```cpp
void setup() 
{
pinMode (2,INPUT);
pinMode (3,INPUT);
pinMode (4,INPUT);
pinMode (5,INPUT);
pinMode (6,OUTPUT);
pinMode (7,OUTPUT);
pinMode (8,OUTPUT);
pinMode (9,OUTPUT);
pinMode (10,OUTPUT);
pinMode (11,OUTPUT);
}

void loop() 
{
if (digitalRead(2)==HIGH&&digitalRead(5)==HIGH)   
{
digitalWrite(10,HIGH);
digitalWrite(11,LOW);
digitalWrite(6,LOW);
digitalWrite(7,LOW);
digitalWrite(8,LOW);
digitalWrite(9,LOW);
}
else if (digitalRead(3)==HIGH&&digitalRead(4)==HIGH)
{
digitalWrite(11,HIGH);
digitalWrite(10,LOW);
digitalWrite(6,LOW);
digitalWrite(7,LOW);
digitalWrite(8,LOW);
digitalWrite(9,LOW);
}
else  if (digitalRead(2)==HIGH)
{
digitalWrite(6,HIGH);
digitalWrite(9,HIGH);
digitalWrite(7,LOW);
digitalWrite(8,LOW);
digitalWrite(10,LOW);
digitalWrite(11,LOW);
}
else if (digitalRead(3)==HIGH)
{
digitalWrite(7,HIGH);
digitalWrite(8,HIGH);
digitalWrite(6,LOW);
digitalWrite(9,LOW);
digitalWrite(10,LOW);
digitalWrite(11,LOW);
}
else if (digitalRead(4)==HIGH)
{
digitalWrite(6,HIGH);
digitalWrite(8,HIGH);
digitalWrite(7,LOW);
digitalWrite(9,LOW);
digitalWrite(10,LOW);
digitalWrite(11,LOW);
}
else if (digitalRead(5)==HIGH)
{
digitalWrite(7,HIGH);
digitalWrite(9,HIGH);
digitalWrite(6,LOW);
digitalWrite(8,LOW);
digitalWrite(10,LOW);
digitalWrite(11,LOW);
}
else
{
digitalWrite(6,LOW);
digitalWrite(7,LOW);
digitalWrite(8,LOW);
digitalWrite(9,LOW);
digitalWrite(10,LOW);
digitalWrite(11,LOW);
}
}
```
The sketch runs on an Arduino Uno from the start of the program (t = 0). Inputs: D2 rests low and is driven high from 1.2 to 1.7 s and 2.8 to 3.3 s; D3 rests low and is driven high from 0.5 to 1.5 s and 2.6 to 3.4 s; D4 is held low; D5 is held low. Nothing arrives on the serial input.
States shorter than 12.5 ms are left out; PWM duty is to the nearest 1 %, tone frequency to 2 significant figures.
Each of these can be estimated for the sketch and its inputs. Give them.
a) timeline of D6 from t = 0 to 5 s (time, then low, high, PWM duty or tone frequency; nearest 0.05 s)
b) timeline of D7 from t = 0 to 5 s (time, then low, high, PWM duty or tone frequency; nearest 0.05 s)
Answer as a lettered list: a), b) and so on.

a) 0 s low; 1.2 s high; 1.7 s low; 2.8 s high; 3.3 s low
b) 0 s low; 0.5 s high; 1.2 s low; 2.6 s high; 2.8 s low; 3.3 s high; 3.4 s low
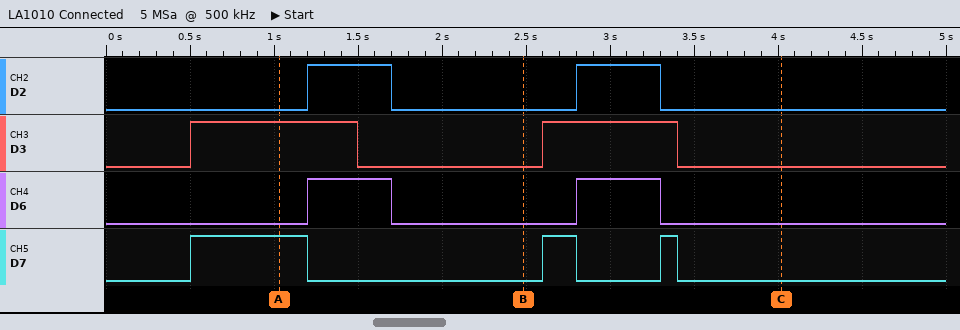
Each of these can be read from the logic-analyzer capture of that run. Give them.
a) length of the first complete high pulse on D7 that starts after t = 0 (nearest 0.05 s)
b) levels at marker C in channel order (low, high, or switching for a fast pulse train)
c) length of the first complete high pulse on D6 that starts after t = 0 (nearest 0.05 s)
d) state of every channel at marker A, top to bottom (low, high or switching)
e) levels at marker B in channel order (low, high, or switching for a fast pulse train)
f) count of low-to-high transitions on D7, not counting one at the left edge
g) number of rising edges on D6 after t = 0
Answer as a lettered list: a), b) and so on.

a) 0.70 s
b) D2 low, D3 low, D6 low, D7 low
c) 0.50 s
d) D2 low, D3 high, D6 low, D7 high
e) D2 low, D3 low, D6 low, D7 low
f) 3
g) 2
